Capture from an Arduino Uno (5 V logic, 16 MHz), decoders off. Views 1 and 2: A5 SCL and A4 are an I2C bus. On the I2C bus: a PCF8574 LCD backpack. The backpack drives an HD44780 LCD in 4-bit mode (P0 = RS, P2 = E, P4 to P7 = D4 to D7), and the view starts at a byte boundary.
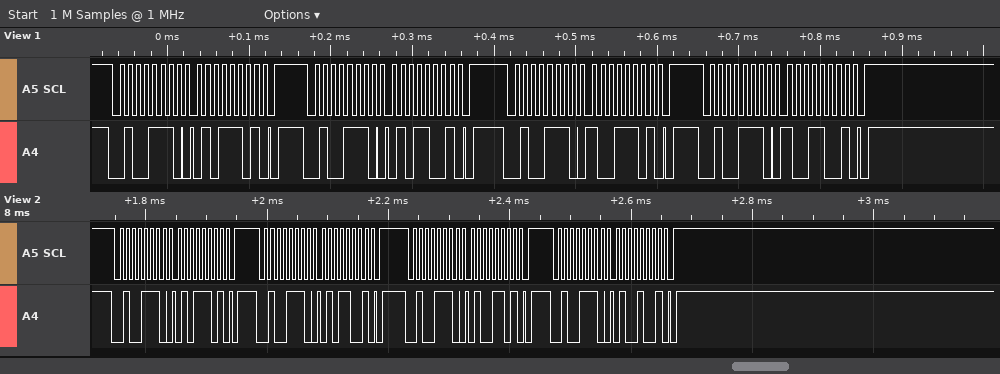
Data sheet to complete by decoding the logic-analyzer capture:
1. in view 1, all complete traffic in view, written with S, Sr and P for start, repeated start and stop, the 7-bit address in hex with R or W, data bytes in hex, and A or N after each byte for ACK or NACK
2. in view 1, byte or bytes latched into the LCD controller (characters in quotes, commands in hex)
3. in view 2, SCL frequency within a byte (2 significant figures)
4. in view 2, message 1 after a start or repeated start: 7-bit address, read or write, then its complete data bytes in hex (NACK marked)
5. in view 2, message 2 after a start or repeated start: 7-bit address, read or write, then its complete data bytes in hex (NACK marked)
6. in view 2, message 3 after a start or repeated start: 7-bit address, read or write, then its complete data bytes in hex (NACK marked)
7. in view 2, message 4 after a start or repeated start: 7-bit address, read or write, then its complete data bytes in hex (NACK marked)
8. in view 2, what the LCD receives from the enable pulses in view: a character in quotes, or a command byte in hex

S 27W A 5D A P S 27W A 59 A P S 27W A 9D A P S 27W A 99 A P
'Y'
100 kHz
0x27 write: 5D
0x27 write: 59
0x27 write: 4D
0x27 write: 49
'T'
